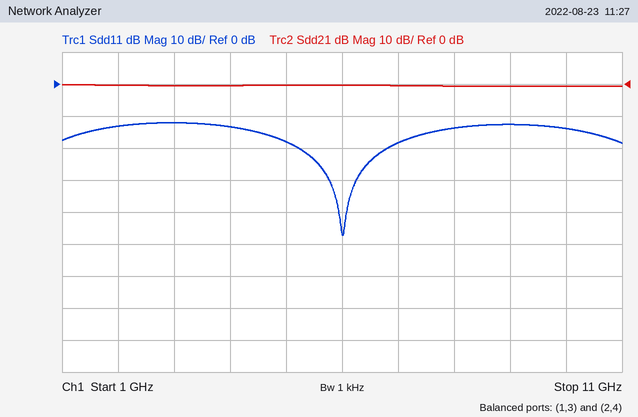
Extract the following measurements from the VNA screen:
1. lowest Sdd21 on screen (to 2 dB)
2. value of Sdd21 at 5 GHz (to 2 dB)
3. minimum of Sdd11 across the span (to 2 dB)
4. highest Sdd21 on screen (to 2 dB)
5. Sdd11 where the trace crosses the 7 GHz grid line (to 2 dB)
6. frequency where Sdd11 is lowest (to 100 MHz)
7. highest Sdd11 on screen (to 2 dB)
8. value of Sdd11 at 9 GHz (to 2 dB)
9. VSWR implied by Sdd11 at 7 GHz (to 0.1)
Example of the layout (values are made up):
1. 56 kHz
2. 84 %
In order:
1. 0 dB
2. 0 dB
3. -48 dB
4. 0 dB
5. -18 dB
6. 6.0 GHz
7. -12 dB
8. -12 dB
9. 1.3
